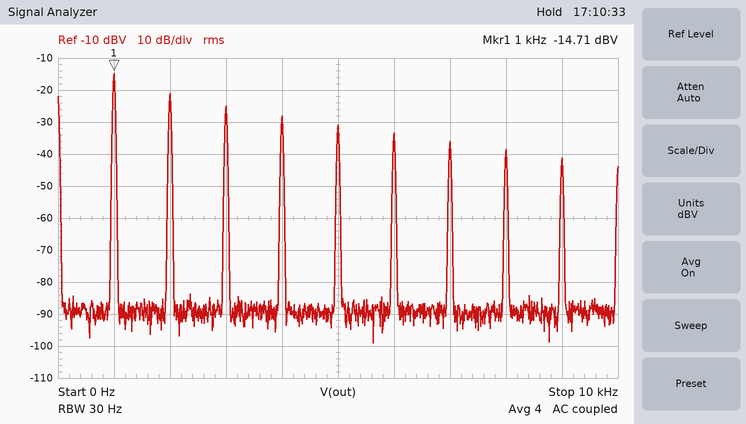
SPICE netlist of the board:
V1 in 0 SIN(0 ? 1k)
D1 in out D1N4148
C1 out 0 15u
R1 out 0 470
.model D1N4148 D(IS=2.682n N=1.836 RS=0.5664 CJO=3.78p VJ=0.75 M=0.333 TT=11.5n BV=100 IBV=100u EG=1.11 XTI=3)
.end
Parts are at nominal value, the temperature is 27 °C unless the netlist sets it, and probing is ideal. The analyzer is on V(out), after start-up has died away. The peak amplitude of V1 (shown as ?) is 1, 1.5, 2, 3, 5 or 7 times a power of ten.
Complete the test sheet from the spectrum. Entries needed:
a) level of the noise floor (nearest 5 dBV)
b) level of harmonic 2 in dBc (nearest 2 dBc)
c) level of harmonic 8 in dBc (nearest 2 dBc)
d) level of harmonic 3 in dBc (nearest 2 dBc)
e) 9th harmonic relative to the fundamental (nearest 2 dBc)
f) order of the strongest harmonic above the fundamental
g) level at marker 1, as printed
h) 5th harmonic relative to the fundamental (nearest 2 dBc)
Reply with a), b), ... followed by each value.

a) -90 dBV
b) -6 dBc
c) -24 dBc
d) -10 dBc
e) -26 dBc
f) 2
g) -14.71 dBV
h) -16 dBc
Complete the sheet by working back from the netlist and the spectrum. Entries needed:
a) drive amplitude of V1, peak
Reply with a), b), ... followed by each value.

a) 7 V
